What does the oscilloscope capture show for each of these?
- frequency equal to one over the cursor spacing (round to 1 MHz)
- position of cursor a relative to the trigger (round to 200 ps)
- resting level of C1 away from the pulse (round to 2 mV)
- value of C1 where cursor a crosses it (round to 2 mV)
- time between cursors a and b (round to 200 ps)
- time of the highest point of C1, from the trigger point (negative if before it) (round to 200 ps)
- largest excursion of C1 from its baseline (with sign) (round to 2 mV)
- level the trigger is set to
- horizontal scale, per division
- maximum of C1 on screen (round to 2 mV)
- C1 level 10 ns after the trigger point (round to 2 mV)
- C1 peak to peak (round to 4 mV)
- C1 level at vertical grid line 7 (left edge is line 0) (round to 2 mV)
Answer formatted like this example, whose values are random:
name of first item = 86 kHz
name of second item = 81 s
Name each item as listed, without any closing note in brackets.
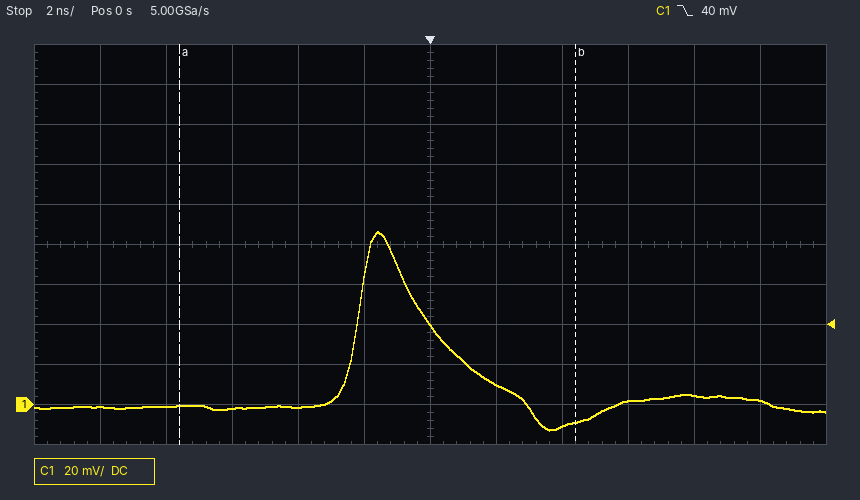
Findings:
frequency equal to one over the cursor spacing = 83 MHz
position of cursor a relative to the trigger = -7.6 ns
resting level of C1 away from the pulse = -2 mV
value of C1 where cursor a crosses it = 0 mV
time between cursors a and b = 12.0 ns
time of the highest point of C1, from the trigger point (negative if before it) = -1.6 ns
largest excursion of C1 from its baseline (with sign) = +88 mV
level the trigger is set to = 40 mV
horizontal scale, per division = 2 ns
maximum of C1 on screen = 86 mV
C1 level 10 ns after the trigger point = 2 mV
C1 peak to peak = 100 mV
C1 level at vertical grid line 7 (left edge is line 0) = 10 mV
